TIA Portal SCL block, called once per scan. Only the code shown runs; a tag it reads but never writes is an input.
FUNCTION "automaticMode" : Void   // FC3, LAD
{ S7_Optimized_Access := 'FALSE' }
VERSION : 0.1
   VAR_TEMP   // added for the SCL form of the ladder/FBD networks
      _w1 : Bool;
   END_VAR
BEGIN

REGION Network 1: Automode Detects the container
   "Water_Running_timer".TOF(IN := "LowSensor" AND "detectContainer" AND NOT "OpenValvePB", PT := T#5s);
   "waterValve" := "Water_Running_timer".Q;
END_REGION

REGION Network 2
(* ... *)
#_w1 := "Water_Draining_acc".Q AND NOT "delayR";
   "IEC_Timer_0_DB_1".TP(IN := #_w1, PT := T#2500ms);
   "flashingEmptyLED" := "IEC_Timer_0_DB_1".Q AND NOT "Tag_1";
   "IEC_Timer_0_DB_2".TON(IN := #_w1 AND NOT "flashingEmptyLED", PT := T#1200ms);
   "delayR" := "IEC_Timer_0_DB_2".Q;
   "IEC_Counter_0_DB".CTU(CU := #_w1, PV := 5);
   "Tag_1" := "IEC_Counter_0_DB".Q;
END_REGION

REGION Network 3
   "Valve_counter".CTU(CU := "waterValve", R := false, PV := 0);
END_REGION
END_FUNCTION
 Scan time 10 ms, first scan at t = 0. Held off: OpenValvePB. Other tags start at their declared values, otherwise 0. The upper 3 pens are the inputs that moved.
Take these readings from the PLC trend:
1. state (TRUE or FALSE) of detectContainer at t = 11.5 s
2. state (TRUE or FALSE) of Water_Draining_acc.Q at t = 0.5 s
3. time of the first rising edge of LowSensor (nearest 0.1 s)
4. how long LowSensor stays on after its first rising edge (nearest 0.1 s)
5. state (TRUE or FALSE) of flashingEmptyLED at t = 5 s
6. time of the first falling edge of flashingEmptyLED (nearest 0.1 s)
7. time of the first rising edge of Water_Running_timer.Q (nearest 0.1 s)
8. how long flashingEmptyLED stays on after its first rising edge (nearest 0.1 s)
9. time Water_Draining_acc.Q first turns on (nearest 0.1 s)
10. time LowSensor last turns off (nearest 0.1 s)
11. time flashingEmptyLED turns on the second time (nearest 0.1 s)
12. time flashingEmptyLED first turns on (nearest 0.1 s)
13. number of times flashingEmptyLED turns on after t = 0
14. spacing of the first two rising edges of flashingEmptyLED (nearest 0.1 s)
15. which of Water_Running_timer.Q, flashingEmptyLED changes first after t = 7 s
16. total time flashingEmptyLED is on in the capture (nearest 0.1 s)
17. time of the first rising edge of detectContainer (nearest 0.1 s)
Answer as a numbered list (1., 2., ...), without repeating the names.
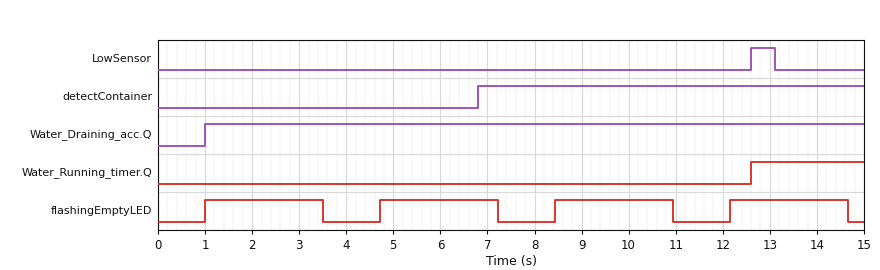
1. TRUE
2. FALSE
3. 12.6 s
4. 0.5 s
5. TRUE
6. 3.5 s
7. 12.6 s
8. 2.5 s
9. 1.0 s
10. 13.1 s
11. 4.7 s
12. 1.0 s
13. 4
14. 3.7 s
15. flashingEmptyLED
16. 10.0 s
17. 6.8 s
